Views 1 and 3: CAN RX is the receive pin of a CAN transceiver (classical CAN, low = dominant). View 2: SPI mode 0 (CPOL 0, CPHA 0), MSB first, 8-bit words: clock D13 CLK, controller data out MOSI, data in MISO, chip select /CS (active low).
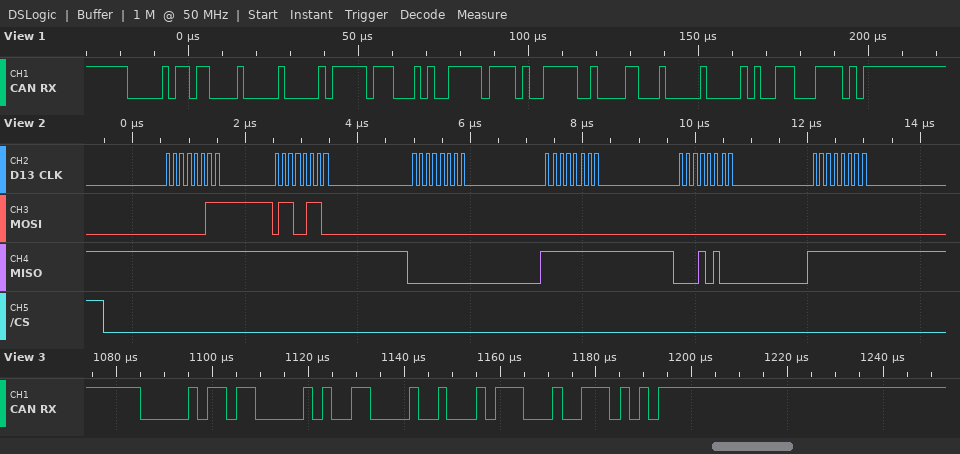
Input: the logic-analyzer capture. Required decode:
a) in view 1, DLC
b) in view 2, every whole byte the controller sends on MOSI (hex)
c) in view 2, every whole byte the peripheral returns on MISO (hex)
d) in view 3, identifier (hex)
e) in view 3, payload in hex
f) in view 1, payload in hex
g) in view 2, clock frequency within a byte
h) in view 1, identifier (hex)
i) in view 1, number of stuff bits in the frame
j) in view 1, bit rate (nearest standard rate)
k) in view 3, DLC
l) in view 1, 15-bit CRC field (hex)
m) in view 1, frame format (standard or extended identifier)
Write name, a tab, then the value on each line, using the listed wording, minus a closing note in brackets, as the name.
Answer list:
in view 1, DLC	8
in view 2, every whole byte the controller sends on MOSI	03 66 00 00 00 00
in view 2, every whole byte the peripheral returns on MISO	FF FF 00 FF 14 FF
in view 3, identifier	0x036
in view 3, payload in hex	61 22
in view 1, payload in hex	00 FF 14 FF A7 D0 C4 00
in view 2, clock frequency within a byte	8 MHz
in view 1, identifier	0x036
in view 1, number of stuff bits in the frame	8
in view 1, bit rate	500 kbit/s
in view 3, DLC	2
in view 1, 15-bit CRC field	0x271E
in view 1, frame format	standard
